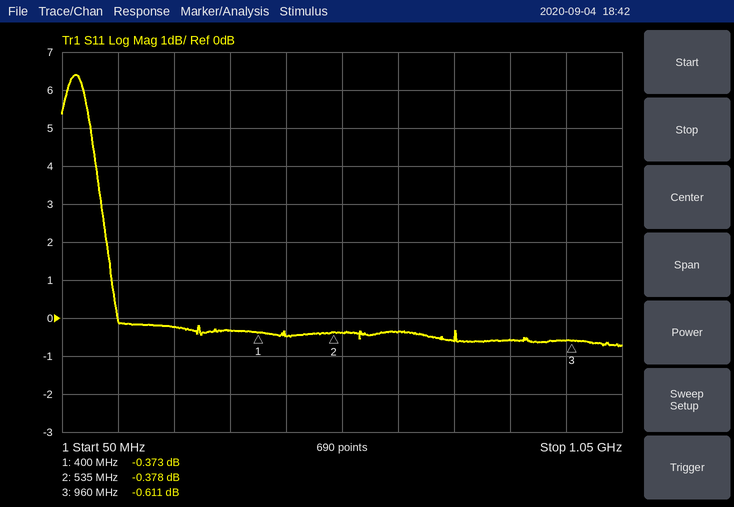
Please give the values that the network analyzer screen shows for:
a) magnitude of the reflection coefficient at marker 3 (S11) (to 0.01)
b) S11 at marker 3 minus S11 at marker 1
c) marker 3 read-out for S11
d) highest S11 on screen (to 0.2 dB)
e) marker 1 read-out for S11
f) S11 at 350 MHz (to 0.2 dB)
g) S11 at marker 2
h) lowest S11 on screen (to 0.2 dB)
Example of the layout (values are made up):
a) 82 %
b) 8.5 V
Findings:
a) 0.93
b) -0.238 dB
c) -0.611 dB
d) 6.4 dB
e) -0.373 dB
f) -0.4 dB
g) -0.378 dB
h) -0.8 dB
